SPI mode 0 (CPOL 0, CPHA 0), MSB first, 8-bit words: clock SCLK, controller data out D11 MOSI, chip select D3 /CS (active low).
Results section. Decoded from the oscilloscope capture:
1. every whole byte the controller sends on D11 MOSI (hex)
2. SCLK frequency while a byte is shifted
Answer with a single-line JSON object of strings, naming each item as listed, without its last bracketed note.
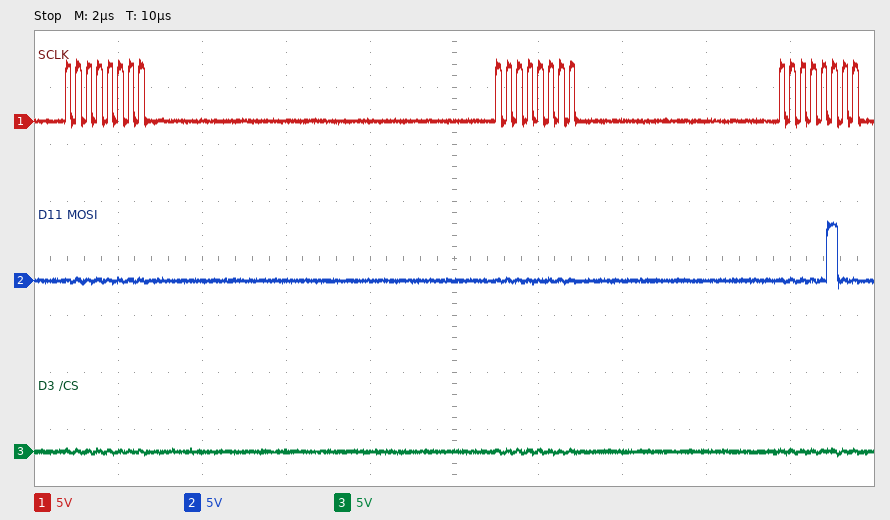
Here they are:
{"every whole byte the controller sends on D11 MOSI": "00 00 04", "SCLK frequency while a byte is shifted": "4 MHz"}
